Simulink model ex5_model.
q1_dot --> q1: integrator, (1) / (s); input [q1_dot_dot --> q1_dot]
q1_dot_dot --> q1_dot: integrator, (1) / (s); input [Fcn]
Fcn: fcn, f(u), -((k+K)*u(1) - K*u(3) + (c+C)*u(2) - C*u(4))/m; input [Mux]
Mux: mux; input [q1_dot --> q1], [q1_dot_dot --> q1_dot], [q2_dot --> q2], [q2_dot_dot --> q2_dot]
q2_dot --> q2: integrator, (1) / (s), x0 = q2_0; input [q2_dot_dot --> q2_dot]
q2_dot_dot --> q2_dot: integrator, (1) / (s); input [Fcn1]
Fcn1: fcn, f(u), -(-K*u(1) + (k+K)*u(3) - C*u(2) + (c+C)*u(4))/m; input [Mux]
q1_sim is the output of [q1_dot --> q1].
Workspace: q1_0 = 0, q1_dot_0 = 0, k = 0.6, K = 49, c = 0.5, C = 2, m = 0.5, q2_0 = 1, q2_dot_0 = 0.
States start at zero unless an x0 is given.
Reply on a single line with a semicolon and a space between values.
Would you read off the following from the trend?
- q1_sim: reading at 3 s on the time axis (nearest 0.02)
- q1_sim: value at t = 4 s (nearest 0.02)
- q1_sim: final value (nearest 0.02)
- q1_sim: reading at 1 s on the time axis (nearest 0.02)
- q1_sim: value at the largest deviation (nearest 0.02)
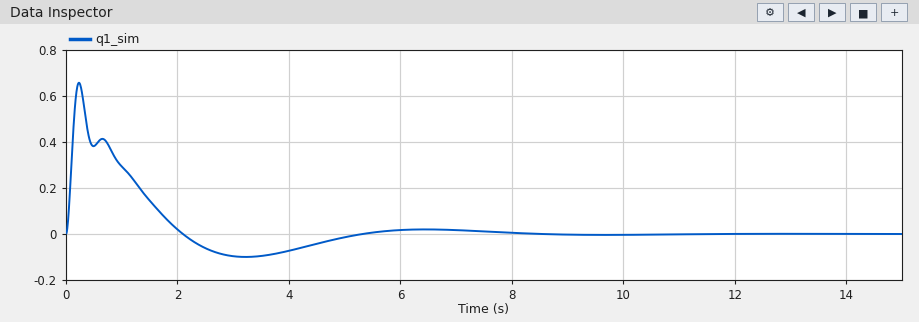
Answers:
-0.10; -0.08; 0.00; 0.30; 0.66
